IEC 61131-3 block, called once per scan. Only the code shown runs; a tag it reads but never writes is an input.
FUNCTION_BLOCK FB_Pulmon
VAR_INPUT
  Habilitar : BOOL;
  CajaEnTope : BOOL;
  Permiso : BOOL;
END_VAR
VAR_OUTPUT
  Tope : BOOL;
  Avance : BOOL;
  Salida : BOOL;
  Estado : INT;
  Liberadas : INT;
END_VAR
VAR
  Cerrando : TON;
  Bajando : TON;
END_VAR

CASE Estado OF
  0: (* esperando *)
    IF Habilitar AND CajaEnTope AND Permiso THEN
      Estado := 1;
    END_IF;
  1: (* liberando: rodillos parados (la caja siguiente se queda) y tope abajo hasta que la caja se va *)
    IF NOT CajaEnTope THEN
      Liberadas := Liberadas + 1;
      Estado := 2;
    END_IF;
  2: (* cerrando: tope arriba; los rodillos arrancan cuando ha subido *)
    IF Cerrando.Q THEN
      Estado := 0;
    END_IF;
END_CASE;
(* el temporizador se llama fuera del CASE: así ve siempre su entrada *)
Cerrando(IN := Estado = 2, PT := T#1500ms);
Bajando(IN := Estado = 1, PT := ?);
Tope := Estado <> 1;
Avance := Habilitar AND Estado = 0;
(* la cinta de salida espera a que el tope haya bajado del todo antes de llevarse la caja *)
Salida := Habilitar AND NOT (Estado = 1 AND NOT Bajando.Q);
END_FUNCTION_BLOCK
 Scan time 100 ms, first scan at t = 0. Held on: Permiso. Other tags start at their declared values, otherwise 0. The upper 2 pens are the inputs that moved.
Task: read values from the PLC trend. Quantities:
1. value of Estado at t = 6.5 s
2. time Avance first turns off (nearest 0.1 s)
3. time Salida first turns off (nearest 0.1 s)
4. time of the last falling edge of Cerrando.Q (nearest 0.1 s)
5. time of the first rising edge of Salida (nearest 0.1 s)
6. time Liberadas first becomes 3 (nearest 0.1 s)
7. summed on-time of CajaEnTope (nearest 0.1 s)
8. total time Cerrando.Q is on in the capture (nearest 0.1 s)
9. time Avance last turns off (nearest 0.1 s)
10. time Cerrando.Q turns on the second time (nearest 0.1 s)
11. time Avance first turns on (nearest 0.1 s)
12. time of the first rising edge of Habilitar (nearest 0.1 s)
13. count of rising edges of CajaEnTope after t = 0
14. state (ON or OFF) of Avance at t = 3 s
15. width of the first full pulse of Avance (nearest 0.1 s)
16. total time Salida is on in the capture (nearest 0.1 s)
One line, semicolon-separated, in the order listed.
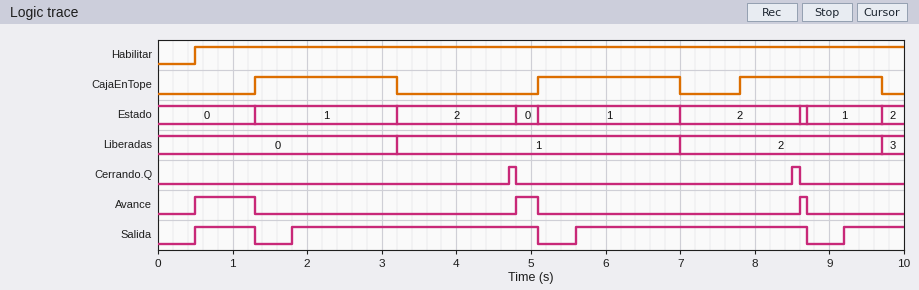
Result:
1; 1.3 s; 1.3 s; 8.6 s; 0.5 s; 9.7 s; 5.7 s; 0.2 s; 8.7 s; 8.5 s; 0.5 s; 0.5 s; 3; OFF; 0.8 s; 8.0 s
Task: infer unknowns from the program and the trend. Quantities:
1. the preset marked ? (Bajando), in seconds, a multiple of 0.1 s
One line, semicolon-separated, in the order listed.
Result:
0.5 s
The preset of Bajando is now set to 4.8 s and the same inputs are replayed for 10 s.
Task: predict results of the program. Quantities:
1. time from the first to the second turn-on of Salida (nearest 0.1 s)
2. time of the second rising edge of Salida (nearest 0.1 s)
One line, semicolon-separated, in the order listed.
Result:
2.7 s; 3.2 s
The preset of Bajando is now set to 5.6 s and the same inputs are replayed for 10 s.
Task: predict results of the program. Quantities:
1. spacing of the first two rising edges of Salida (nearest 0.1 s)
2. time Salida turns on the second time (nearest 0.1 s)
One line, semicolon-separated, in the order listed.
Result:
2.7 s; 3.2 s
